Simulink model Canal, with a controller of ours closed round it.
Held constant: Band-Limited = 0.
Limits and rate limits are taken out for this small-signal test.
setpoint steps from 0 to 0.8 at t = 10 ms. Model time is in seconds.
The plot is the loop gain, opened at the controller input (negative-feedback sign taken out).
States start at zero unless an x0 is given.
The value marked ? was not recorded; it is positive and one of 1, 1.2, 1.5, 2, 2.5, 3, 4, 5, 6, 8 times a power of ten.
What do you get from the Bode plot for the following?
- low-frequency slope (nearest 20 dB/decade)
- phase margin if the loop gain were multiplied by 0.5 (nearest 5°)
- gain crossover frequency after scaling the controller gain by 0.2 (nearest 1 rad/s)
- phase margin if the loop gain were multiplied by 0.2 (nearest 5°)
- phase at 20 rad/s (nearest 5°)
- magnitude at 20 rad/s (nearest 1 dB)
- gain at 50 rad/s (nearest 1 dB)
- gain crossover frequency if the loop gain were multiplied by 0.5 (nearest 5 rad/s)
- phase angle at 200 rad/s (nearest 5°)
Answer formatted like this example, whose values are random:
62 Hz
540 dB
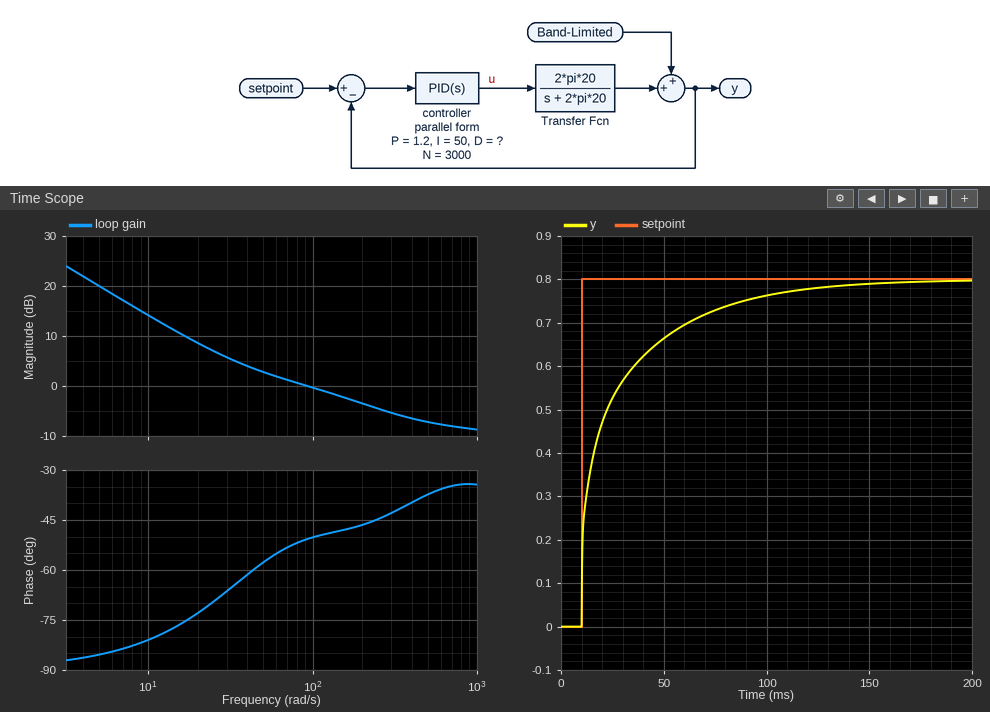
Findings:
-20 dB/decade
115°
10 rad/s
100°
-75°
9 dB
3 dB
30 rad/s
-45°
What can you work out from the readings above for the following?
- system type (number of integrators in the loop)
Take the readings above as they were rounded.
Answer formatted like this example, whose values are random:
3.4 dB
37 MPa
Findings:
1
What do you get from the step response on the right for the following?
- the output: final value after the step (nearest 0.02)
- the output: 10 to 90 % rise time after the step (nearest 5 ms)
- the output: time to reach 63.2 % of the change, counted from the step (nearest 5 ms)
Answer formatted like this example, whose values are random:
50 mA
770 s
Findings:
0.80
60 ms
15 ms
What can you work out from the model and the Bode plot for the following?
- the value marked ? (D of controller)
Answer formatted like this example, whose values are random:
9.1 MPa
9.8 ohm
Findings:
0.0025
